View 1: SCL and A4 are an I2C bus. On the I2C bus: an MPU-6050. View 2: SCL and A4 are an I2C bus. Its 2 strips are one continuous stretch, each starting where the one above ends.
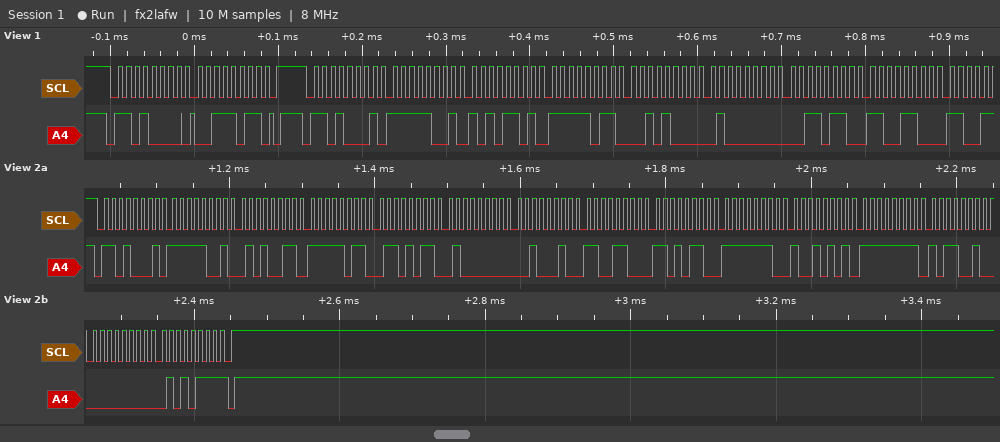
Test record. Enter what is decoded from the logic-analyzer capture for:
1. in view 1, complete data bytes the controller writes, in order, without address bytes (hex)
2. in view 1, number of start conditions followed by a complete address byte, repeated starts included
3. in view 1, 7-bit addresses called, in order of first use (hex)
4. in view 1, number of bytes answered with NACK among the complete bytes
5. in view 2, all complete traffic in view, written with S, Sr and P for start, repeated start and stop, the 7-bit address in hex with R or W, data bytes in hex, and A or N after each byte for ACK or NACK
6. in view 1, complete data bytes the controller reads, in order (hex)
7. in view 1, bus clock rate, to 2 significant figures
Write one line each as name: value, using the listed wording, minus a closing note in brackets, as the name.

in view 1, complete data bytes the controller writes, in order, without address bytes: 3B
in view 1, number of start conditions followed by a complete address byte, repeated starts included: 2
in view 1, 7-bit addresses called, in order of first use: 0x68
in view 1, number of bytes answered with NACK among the complete bytes: 0
in view 2, all complete traffic in view, written with S, Sr and P for start, repeated start and stop, the 7-bit address in hex with R or W, data bytes in hex, and A or N after each byte for ACK or NACK: S 68R A F9 A 53 A FB A 6B A 40 A 22 A CC A D6 A FE A 95 A FF A B2 A 00 A 57 N P
in view 1, complete data bytes the controller reads, in order: F9 AD FB 28 40 36 CC
in view 1, bus clock rate, to 2 significant figures: 100 kHz
